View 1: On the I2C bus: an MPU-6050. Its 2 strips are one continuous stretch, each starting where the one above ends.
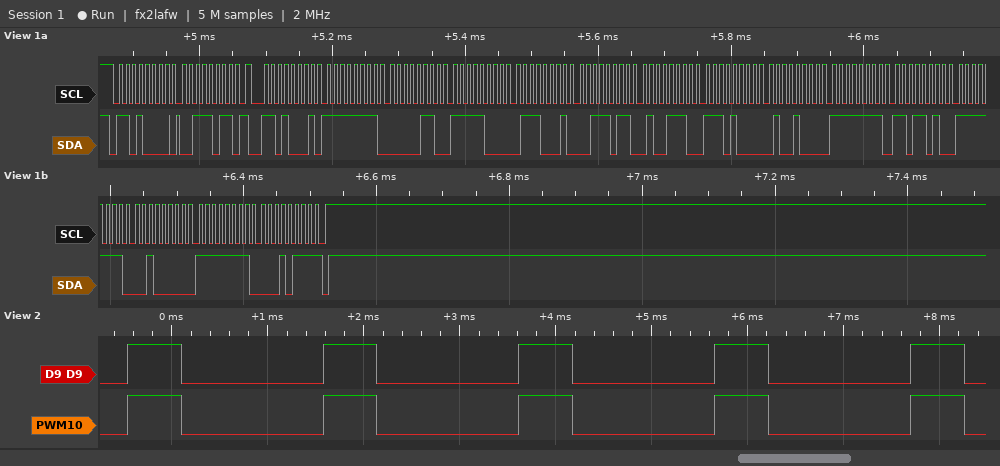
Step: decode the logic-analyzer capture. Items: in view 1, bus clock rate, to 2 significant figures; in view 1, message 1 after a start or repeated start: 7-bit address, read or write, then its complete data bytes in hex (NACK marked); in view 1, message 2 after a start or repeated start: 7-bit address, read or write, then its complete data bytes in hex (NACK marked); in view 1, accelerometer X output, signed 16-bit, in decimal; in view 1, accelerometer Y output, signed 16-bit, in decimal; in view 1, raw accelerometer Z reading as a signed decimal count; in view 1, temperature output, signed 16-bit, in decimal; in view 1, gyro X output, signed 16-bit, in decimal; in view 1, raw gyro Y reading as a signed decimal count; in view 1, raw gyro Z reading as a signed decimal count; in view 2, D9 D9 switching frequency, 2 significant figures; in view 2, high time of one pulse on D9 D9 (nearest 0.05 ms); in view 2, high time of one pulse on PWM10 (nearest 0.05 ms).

100 kHz
0x68 write: 3B
0x68 read: FF 06 F8 71 3B 4E E8 48 FF DA FF 20 FF 17 NACK
-250
-1935
15182
-6072
-38
-224
-233
490 Hz
0.55 ms
0.55 ms
